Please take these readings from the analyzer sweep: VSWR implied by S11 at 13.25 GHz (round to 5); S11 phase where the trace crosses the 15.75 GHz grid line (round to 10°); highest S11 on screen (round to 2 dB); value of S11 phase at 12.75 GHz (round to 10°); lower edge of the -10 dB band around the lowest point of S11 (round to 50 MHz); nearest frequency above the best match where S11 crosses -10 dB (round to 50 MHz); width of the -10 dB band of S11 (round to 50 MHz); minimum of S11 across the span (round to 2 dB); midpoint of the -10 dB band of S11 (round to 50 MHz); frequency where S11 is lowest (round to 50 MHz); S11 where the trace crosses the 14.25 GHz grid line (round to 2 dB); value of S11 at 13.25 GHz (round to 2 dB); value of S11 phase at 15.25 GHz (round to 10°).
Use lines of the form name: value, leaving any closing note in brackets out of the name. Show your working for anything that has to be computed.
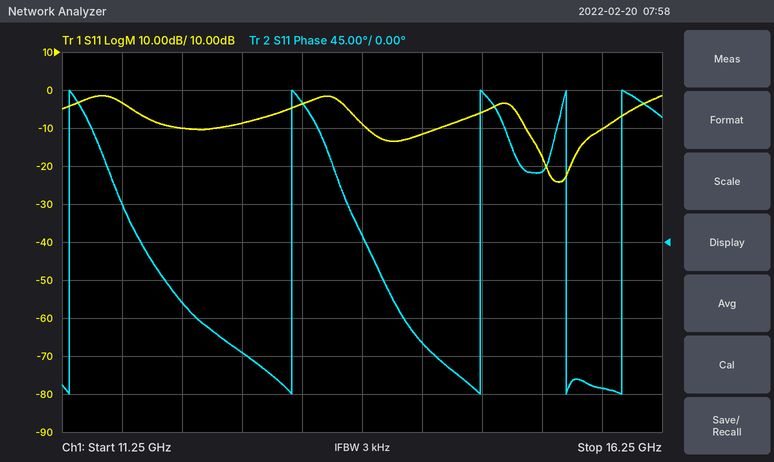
VSWR implied by S11 at 13.25 GHz: |Γ| = 10^(-4/20) = 0.6310; VSWR = (1 + 0.6310)/(1 − 0.6310) ≈ 4.42, so 5 to the nearest 5
S11 phase where the trace crosses the 15.75 GHz grid line: -170°
highest S11 on screen: -2 dB
value of S11 phase at 12.75 GHz: -130°
lower edge of the -10 dB band around the lowest point of S11: 15.10 GHz
nearest frequency above the best match where S11 crosses -10 dB: 15.75 GHz
width of the -10 dB band of S11: 15.75 GHz − 15.10 GHz = 650 MHz
minimum of S11 across the span: -24 dB
midpoint of the -10 dB band of S11: 15.45 GHz
frequency where S11 is lowest: 15.40 GHz
S11 where the trace crosses the 14.25 GHz grid line: -12 dB
value of S11 at 13.25 GHz: -4 dB
value of S11 phase at 15.25 GHz: 80°
